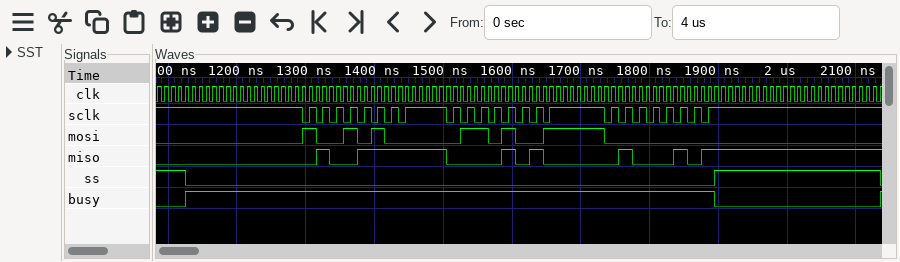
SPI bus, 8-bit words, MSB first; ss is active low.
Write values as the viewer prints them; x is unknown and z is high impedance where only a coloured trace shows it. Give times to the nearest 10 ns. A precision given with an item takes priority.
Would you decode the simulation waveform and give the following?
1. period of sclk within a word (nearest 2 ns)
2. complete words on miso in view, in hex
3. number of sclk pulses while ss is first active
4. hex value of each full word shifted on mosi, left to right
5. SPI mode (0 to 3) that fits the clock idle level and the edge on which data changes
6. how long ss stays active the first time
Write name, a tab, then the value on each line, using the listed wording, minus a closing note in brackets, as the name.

period of sclk within a word	20 ns
complete words on miso in view, in hex	4F, 0A, 45
number of sclk pulses while ss is first active	24
hex value of each full word shifted on mosi, left to right	94, 69, 00
SPI mode (0 to 3) that fits the clock idle level and the edge on which data changes	3
how long ss stays active the first time	770 ns
